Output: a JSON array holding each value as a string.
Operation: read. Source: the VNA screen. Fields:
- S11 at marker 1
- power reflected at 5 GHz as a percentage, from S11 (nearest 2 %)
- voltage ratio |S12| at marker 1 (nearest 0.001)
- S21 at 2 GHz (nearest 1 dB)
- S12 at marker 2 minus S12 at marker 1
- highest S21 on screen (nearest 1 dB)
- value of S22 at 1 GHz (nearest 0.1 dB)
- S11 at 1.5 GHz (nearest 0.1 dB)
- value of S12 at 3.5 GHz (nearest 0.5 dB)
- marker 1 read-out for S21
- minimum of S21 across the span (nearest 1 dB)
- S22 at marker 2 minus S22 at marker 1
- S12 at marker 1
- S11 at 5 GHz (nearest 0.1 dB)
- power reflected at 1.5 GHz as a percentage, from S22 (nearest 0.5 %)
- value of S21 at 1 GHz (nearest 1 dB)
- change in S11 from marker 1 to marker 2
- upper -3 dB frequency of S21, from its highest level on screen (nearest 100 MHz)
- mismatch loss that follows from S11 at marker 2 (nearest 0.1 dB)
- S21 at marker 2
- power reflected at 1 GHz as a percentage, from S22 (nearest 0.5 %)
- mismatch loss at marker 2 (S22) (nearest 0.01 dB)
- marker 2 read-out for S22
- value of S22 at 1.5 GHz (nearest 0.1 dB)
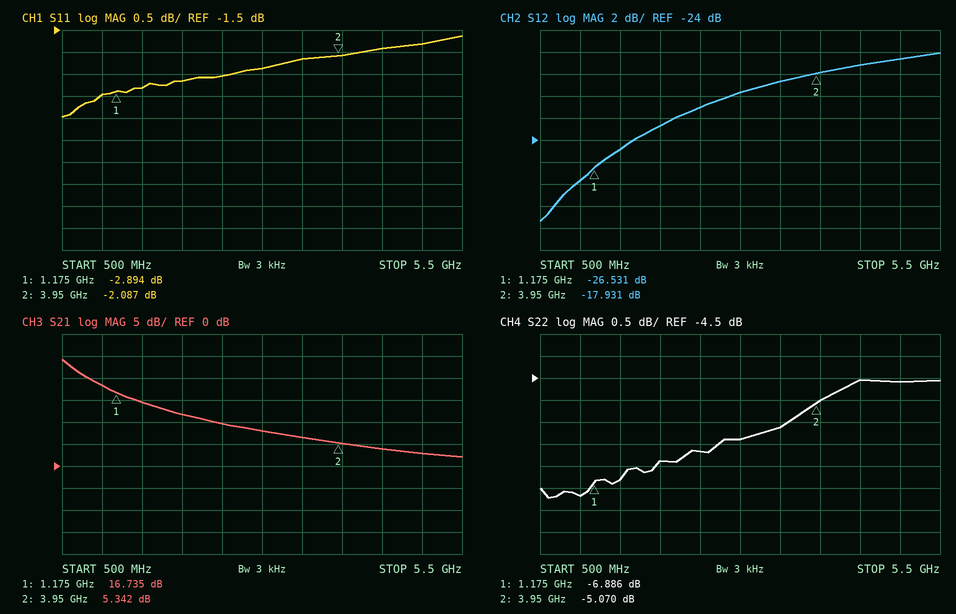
["-2.894 dB", "66 %", "0.047", "12 dB", "8.600 dB", "24 dB", "-7.2 dB", "-2.8 dB", "-18.5 dB", "16.735 dB", "2 dB", "1.816 dB", "-26.531 dB", "-1.8 dB", "21.0 %", "18 dB", "0.807 dB", "700 MHz", "4.2 dB", "5.342 dB", "19.0 %", "1.62 dB", "-5.070 dB", "-6.8 dB"]
